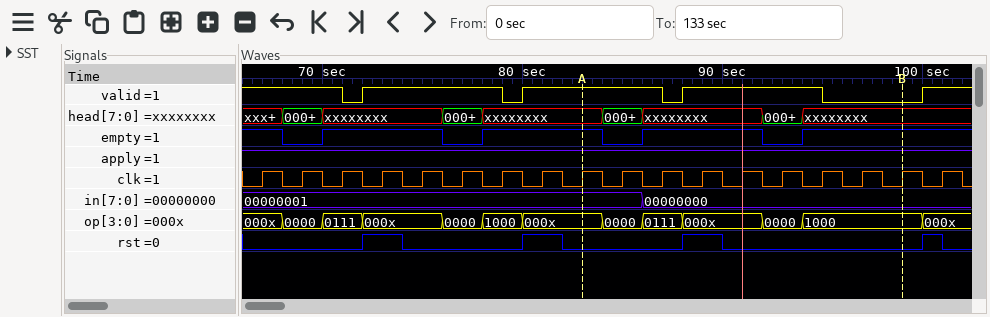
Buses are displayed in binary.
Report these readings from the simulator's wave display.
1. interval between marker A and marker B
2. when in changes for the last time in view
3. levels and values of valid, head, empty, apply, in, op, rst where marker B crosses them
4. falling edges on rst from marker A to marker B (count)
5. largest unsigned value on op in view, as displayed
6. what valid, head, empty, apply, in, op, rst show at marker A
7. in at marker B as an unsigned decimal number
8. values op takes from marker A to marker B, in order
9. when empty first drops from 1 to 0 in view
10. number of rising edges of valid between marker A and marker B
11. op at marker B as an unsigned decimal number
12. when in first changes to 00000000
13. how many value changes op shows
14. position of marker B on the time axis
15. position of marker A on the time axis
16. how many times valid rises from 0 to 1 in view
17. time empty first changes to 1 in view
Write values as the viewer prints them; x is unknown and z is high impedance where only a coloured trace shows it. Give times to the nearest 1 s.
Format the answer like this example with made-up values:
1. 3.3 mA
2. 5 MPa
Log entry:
1. 16 s
2. 86 s
3. valid=0, head=xxxxxxxx, empty=1, apply=1, in=00000000, op=1000, rst=0
4. 1
5. 1000
6. valid=1, head=xxxxxxxx, empty=1, apply=1, in=00000001, op=000x, rst=0
7. 0
8. 000x, 0000, 0111, 000x, 0000, 1000
9. 68 s
10. 1
11. 8
12. 86 s
13. 12
14. 99 s
15. 83 s
16. 4
17. 70 s
